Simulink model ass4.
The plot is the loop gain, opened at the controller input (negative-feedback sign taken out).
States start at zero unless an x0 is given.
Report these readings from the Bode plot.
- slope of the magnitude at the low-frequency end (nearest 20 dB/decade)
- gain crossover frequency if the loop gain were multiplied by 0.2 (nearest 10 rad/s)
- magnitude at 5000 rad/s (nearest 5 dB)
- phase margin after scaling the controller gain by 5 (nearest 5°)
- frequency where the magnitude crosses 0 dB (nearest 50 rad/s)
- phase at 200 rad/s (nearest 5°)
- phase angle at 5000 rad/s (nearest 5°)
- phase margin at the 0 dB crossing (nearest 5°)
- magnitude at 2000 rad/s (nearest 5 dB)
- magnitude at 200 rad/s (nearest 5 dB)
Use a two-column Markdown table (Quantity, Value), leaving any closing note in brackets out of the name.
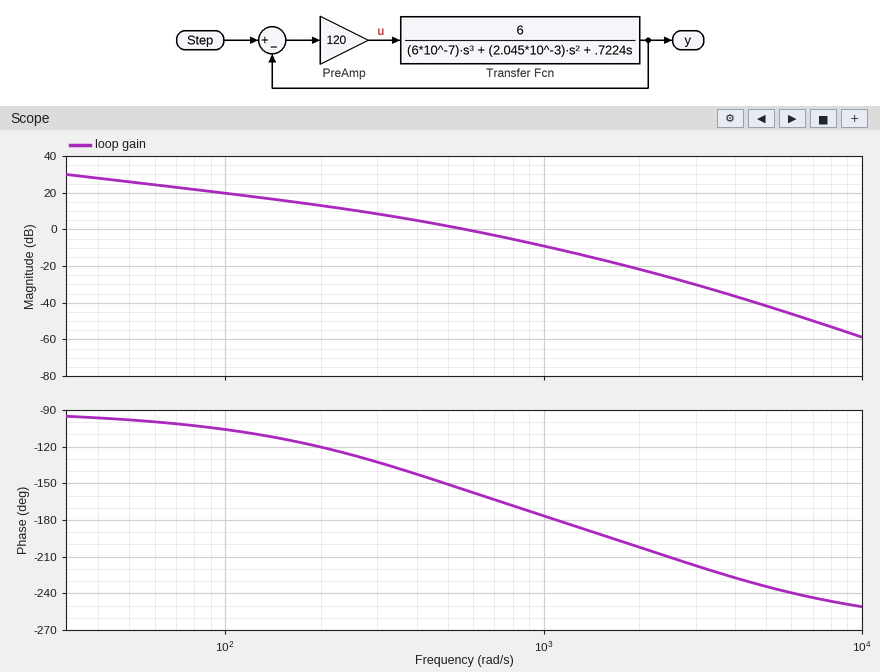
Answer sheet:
| Quantity | Value |
|---|---|
| slope of the magnitude at the low-frequency end | -20 dB/decade |
| gain crossover frequency if the loop gain were multiplied by 0.2 | 180 rad/s |
| magnitude at 5000 rad/s | -40 dB |
| phase margin after scaling the controller gain by 5 | -5° |
| frequency where the magnitude crosses 0 dB | 550 rad/s |
| phase at 200 rad/s | -120° |
| phase angle at 5000 rad/s | -235° |
| phase margin at the 0 dB crossing | 25° |
| magnitude at 2000 rad/s | -20 dB |
| magnitude at 200 rad/s | 15 dB |
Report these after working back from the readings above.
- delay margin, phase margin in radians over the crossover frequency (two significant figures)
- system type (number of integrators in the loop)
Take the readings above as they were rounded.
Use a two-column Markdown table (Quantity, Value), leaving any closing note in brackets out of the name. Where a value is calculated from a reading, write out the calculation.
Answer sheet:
| Quantity | Value |
|---|---|
| delay margin, phase margin in radians over the crossover frequency | 25 × π / 180 / 550 = 0.00079 s |
| system type | 1 |
